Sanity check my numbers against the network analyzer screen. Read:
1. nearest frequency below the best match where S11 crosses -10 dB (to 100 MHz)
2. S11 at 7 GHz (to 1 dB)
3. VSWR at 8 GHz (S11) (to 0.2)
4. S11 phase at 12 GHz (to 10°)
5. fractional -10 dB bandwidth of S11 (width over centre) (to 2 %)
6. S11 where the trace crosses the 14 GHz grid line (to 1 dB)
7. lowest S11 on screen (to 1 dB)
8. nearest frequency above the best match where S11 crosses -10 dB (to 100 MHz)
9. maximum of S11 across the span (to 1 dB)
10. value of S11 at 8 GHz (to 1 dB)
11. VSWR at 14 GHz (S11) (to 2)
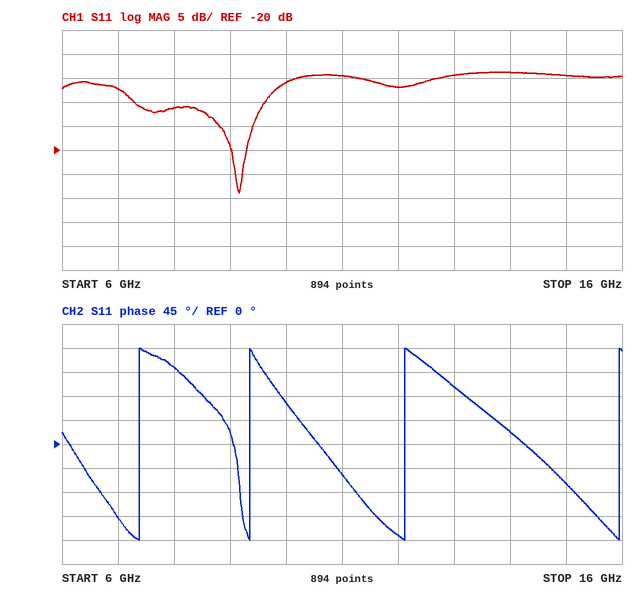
7.3 GHz
-7 dB
1.8
-170°
28 %
-4 dB
-29 dB
9.6 GHz
-4 dB
-11 dB
4
